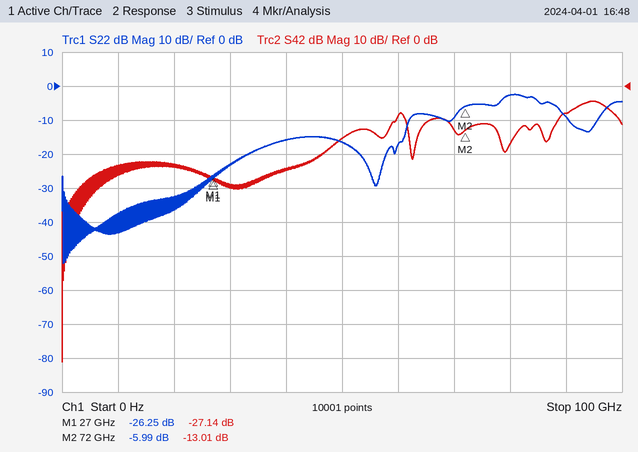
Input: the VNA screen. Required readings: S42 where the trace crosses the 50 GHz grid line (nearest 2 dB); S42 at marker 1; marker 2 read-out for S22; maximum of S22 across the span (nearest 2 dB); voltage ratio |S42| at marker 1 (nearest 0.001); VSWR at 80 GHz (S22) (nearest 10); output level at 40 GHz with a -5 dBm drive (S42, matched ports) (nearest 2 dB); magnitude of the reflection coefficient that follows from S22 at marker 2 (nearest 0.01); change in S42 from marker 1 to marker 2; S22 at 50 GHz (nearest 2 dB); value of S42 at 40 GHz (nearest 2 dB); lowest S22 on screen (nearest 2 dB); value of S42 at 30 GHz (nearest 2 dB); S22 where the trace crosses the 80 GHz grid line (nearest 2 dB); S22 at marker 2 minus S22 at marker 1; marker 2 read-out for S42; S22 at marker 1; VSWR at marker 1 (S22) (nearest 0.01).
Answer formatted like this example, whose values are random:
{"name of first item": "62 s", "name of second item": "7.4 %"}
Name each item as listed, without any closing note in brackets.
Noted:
{"S42 where the trace crosses the 50 GHz grid line": "-16 dB", "S42 at marker 1": "-27.14 dB", "marker 2 read-out for S22": "-5.99 dB", "maximum of S22 across the span": "-2 dB", "voltage ratio |S42| at marker 1": "0.044", "VSWR at 80 GHz (S22)": "10", "output level at 40 GHz with a -5 dBm drive (S42, matched ports)": "-30 dBm", "magnitude of the reflection coefficient that follows from S22 at marker 2": "0.50", "change in S42 from marker 1 to marker 2": "14.13 dB", "S22 at 50 GHz": "-16 dB", "value of S42 at 40 GHz": "-24 dB", "lowest S22 on screen": "-52 dB", "value of S42 at 30 GHz": "-30 dB", "S22 where the trace crosses the 80 GHz grid line": "-2 dB", "S22 at marker 2 minus S22 at marker 1": "20.26 dB", "marker 2 read-out for S42": "-13.01 dB", "S22 at marker 1": "-26.25 dB", "VSWR at marker 1 (S22)": "1.10"}
